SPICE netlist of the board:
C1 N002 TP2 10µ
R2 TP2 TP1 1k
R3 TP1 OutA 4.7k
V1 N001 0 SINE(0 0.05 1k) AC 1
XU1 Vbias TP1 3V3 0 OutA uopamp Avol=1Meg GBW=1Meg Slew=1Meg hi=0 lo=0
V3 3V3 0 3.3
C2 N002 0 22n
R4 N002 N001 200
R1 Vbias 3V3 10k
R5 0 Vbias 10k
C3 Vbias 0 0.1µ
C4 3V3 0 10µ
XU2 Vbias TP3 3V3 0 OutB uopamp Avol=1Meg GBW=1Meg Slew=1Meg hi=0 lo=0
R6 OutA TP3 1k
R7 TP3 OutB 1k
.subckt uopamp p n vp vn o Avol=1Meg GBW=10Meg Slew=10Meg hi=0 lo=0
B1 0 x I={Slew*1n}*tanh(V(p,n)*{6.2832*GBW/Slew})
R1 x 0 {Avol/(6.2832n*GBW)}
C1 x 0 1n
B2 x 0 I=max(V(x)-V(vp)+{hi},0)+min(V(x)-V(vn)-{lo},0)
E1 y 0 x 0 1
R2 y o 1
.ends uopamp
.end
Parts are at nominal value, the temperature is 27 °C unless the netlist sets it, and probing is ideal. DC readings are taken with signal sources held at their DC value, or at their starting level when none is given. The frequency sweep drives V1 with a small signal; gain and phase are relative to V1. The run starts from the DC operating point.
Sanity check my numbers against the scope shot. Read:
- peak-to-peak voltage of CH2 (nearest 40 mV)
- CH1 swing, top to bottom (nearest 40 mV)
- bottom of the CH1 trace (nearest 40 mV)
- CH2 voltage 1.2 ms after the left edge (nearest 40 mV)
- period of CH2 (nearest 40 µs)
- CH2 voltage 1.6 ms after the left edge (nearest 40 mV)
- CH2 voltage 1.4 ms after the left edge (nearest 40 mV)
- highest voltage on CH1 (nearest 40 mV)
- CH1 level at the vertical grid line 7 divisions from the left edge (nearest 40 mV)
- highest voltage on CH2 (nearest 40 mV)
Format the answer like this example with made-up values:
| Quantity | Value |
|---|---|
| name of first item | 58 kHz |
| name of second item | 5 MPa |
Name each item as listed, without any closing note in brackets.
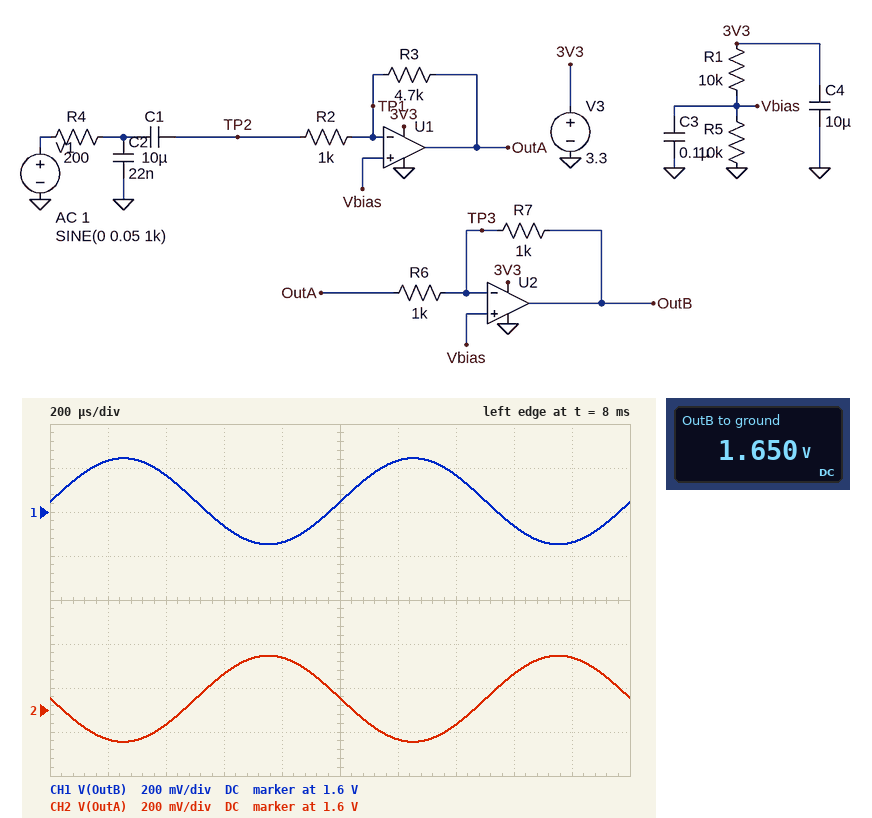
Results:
| Quantity | Value |
|---|---|
| peak-to-peak voltage of CH2 | 400 mV |
| CH1 swing, top to bottom | 400 mV |
| bottom of the CH1 trace | 1.44 V |
| CH2 voltage 1.2 ms after the left edge | 1.48 V |
| period of CH2 | 1.00 ms |
| CH2 voltage 1.6 ms after the left edge | 1.76 V |
| CH2 voltage 1.4 ms after the left edge | 1.52 V |
| highest voltage on CH1 | 1.84 V |
| CH1 level at the vertical grid line 7 divisions from the left edge | 1.76 V |
| highest voltage on CH2 | 1.84 V |
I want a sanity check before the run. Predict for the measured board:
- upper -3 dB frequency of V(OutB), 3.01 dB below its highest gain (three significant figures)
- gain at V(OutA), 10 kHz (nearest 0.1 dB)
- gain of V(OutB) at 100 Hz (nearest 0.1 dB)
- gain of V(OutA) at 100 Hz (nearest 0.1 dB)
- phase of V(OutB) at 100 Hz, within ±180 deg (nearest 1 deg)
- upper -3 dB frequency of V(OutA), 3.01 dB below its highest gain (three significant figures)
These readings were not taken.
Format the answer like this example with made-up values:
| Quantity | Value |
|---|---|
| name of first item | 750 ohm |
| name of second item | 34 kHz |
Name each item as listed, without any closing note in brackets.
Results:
| Quantity | Value |
|---|---|
| upper -3 dB frequency of V(OutB), 3.01 dB below its highest gain | 42.4 kHz |
| gain at V(OutA), 10 kHz | 11.6 dB |
| gain of V(OutB) at 100 Hz | 11.8 dB |
| gain of V(OutA) at 100 Hz | 11.8 dB |
| phase of V(OutB) at 100 Hz, within ±180 deg | 7 deg |
| upper -3 dB frequency of V(OutA), 3.01 dB below its highest gain | 42.7 kHz |
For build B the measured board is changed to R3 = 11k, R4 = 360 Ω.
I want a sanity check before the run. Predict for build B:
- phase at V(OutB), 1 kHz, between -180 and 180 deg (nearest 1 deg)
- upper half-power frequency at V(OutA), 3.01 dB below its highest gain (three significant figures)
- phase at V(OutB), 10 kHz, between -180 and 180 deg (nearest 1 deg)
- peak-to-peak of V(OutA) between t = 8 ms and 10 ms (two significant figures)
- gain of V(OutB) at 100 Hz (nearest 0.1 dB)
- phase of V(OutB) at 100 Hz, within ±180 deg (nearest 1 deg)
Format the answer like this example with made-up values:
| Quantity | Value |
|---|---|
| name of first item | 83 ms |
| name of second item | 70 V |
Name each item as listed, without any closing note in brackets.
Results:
| Quantity | Value |
|---|---|
| phase at V(OutB), 1 kHz, between -180 and 180 deg | -2 deg |
| upper half-power frequency at V(OutA), 3.01 dB below its highest gain | 27.2 kHz |
| phase at V(OutB), 10 kHz, between -180 and 180 deg | -27 deg |
| peak-to-peak of V(OutA) between t = 8 ms and 10 ms | 810 mV |
| gain of V(OutB) at 100 Hz | 18.1 dB |
| phase of V(OutB) at 100 Hz, within ±180 deg | 6 deg |
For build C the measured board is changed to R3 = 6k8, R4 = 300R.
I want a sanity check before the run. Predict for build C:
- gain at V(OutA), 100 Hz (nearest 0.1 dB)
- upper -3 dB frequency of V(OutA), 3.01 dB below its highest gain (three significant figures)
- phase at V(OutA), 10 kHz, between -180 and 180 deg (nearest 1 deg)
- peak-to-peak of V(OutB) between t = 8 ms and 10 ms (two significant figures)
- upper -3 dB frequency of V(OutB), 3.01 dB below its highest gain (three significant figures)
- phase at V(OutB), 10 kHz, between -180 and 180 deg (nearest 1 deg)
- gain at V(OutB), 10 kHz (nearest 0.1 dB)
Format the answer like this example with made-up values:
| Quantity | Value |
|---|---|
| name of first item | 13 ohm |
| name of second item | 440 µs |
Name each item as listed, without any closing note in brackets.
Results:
| Quantity | Value |
|---|---|
| gain at V(OutA), 100 Hz | 14.3 dB |
| upper -3 dB frequency of V(OutA), 3.01 dB below its highest gain | 31.4 kHz |
| phase at V(OutA), 10 kHz, between -180 and 180 deg | 159 deg |
| peak-to-peak of V(OutB) between t = 8 ms and 10 ms | 520 mV |
| upper -3 dB frequency of V(OutB), 3.01 dB below its highest gain | 31.3 kHz |
| phase at V(OutB), 10 kHz, between -180 and 180 deg | -22 deg |
| gain at V(OutB), 10 kHz | 14.0 dB |
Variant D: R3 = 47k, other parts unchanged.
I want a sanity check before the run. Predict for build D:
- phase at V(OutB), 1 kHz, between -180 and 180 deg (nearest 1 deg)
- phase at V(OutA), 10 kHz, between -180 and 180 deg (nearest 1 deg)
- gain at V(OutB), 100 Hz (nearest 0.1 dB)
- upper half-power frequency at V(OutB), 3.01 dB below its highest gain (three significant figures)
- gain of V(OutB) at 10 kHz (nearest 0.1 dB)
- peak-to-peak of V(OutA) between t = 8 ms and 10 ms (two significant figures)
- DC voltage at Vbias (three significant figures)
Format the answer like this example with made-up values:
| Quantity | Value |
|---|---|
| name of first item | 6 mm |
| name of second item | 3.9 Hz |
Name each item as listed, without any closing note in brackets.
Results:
| Quantity | Value |
|---|---|
| phase at V(OutB), 1 kHz, between -180 and 180 deg | -3 deg |
| phase at V(OutA), 10 kHz, between -180 and 180 deg | 145 deg |
| gain at V(OutB), 100 Hz | 31.8 dB |
| upper half-power frequency at V(OutB), 3.01 dB below its highest gain | 20.8 kHz |
| gain of V(OutB) at 10 kHz | 31.1 dB |
| peak-to-peak of V(OutA) between t = 8 ms and 10 ms | 3.3 V |
| DC voltage at Vbias | 1.65 V |
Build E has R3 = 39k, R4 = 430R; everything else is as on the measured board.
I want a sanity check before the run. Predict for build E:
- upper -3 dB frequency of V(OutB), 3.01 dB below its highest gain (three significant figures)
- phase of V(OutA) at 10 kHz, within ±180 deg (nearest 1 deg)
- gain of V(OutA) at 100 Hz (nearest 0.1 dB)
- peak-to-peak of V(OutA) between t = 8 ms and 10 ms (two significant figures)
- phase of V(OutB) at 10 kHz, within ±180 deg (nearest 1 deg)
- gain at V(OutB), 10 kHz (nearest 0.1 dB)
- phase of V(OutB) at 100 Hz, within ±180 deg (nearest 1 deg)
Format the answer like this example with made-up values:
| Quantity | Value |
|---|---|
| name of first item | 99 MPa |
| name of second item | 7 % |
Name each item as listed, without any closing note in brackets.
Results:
| Quantity | Value |
|---|---|
| upper -3 dB frequency of V(OutB), 3.01 dB below its highest gain | 19.6 kHz |
| phase of V(OutA) at 10 kHz, within ±180 deg | 140 deg |
| gain of V(OutA) at 100 Hz | 28.7 dB |
| peak-to-peak of V(OutA) between t = 8 ms and 10 ms | 2.7 V |
| phase of V(OutB) at 10 kHz, within ±180 deg | -41 deg |
| gain at V(OutB), 10 kHz | 28.0 dB |
| phase of V(OutB) at 100 Hz, within ±180 deg | 6 deg |
